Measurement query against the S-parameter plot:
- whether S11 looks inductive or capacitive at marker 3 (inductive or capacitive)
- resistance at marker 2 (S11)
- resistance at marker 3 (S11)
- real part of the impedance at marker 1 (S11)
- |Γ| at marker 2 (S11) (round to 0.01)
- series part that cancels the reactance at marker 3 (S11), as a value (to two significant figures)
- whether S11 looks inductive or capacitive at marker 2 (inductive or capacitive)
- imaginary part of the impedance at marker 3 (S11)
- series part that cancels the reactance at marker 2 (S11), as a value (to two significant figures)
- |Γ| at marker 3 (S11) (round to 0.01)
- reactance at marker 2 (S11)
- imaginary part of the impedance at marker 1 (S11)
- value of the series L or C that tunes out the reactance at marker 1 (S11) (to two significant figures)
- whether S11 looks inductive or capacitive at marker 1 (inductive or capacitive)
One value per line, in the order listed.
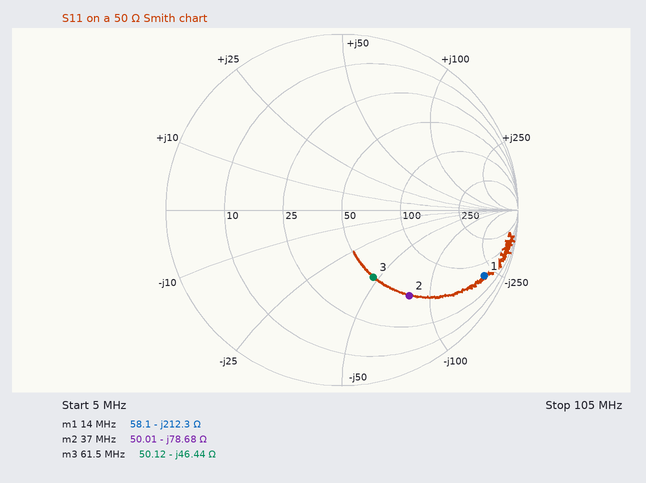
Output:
capacitive
50.01 Ω
50.12 Ω
58.1 Ω
0.62
120 nH
capacitive
-46.44 Ω
340 nH
0.42
-78.68 Ω
-212.3 Ω
2.4 µH
capacitive
